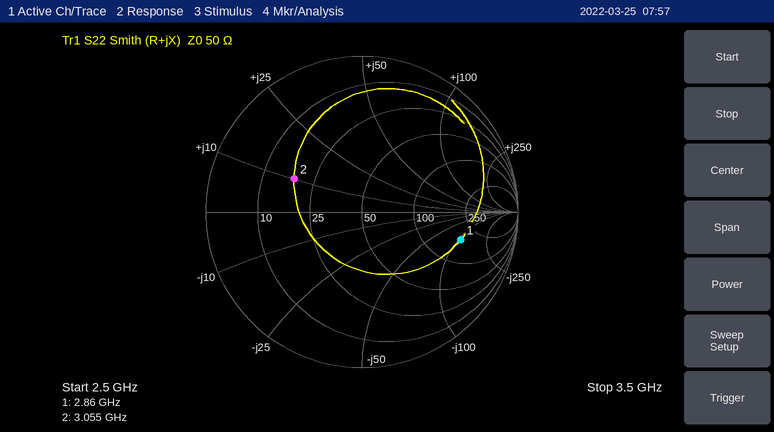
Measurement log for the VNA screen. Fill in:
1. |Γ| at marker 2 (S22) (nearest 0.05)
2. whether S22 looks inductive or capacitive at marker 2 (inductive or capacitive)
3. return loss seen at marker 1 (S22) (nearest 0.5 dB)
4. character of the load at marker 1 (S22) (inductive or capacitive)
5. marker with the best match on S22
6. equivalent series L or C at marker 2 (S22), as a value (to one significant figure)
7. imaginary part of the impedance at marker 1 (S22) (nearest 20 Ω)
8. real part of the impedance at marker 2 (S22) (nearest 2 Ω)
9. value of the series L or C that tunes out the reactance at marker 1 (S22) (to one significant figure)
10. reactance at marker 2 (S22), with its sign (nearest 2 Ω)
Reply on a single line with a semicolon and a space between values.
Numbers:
0.50; inductive; 3.5 dB; capacitive; marker 2; 500 pH; -100 Ω; 18 Ω; 6 nH; +10 Ω
